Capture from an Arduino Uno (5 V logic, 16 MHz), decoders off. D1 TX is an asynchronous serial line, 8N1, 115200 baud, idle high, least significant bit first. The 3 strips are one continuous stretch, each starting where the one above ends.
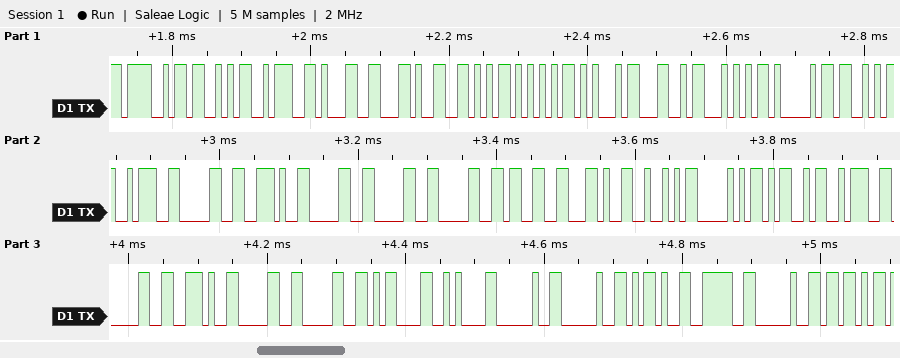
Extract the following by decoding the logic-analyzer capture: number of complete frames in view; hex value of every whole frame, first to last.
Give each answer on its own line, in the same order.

36
4F 53 3A 31 2C 56 55 45 4C 54 41 53 3A 30 2E 30 30 30 33 2C 52 50 4D 3A 30 2E 30 30 0D 0A 20 20 2D 3E 20 5B
